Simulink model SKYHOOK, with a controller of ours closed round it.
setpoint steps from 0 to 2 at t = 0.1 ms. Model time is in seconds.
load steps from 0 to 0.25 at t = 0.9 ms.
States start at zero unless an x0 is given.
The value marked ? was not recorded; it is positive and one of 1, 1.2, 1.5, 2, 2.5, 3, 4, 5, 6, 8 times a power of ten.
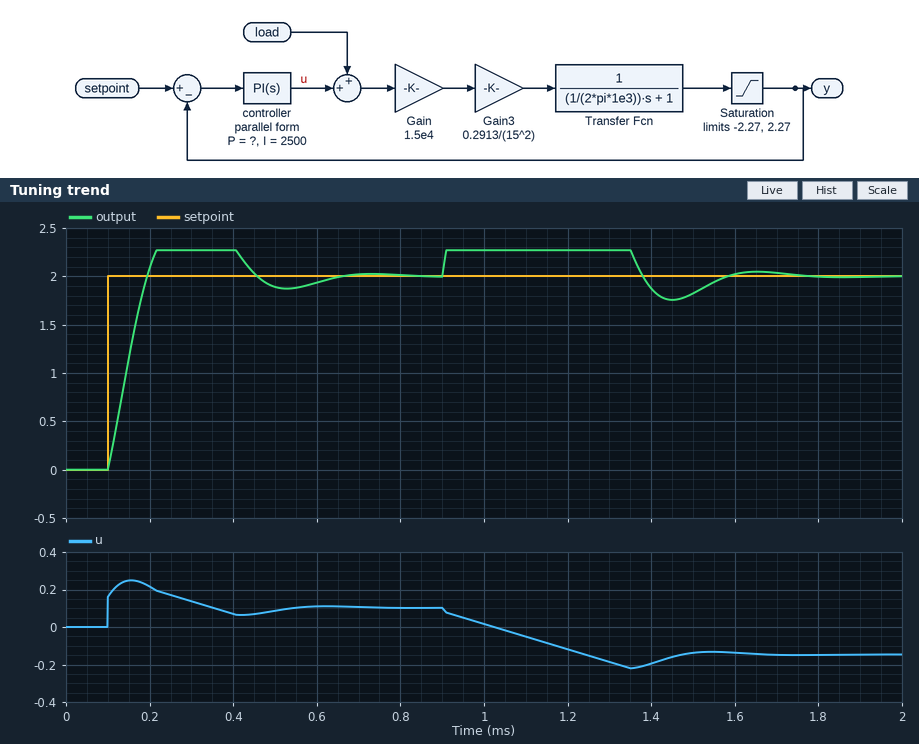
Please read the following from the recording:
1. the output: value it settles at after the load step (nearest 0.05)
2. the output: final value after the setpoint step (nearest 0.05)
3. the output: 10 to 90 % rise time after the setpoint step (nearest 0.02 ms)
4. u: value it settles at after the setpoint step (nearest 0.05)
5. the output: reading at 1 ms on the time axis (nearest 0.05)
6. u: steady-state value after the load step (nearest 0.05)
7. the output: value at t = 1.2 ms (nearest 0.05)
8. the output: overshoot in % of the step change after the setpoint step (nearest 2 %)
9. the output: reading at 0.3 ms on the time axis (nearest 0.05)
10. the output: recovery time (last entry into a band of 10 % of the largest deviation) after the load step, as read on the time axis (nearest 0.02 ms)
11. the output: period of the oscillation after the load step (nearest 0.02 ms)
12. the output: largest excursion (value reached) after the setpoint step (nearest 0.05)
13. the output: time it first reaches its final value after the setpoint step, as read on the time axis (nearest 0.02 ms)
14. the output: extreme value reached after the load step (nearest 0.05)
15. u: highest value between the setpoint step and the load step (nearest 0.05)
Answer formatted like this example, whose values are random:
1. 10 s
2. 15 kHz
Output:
1. 2.00
2. 2.00
3. 0.08 ms
4. 0.10
5. 2.25
6. -0.15
7. 2.25
8. 14 %
9. 2.25
10. 1.72 ms
11. 0.52 ms
12. 2.25
13. 0.20 ms
14. 2.25
15. 0.25
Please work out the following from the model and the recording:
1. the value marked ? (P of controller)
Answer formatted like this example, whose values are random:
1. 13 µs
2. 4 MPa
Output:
1. 0.08
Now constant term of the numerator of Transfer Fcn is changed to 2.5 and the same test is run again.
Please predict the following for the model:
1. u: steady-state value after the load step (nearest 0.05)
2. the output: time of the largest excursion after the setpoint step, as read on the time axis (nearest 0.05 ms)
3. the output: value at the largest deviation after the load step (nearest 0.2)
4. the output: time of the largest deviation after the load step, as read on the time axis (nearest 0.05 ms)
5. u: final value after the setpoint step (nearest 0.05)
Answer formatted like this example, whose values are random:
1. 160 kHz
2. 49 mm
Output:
1. -0.20
2. 0.15 ms
3. 1.6
4. 1.40 ms
5. 0.05
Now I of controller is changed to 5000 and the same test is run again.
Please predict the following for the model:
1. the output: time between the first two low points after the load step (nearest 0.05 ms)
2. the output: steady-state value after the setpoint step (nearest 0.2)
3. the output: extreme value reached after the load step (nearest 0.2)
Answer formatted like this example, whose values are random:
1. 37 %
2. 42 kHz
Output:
1. 0.25 ms
2. 2.0
3. 1.6
